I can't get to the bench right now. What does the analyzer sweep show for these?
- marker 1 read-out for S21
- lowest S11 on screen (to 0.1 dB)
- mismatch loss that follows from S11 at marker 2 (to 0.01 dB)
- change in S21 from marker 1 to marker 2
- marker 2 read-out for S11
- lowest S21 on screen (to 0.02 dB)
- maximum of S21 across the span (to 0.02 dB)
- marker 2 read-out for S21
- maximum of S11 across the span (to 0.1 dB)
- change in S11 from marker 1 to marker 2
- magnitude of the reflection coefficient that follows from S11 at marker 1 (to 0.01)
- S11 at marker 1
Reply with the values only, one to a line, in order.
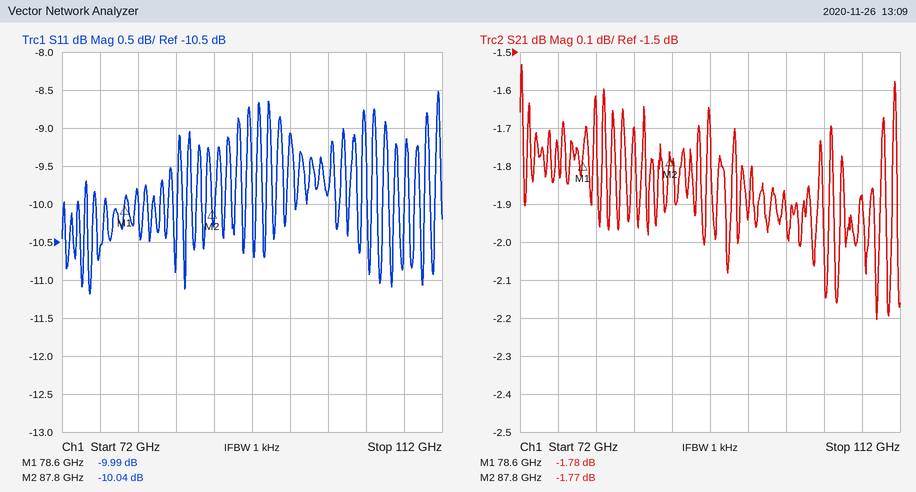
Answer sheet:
-1.78 dB
-11.2 dB
0.45 dB
0.01 dB
-10.04 dB
-2.20 dB
-1.54 dB
-1.77 dB
-8.5 dB
-0.05 dB
0.32
-9.99 dB
